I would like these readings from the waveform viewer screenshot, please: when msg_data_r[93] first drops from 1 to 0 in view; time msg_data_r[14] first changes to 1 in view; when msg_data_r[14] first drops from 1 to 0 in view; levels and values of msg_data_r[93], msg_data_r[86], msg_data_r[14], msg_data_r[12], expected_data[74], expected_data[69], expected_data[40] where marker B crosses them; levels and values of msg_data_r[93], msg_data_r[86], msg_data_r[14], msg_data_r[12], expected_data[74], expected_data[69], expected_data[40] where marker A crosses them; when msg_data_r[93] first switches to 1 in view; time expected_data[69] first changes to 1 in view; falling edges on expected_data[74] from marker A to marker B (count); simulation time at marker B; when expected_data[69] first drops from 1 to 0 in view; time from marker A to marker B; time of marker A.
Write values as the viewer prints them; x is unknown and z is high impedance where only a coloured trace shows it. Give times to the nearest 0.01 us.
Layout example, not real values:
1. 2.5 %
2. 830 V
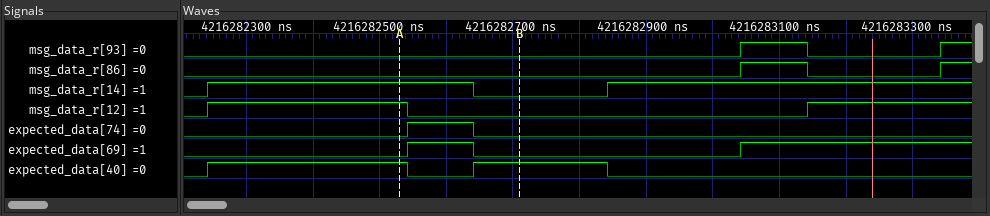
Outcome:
1. 4216283.14 us
2. 4216282.24 us
3. 4216282.64 us
4. msg_data_r[93]=0, msg_data_r[86]=0, msg_data_r[14]=0, msg_data_r[12]=0, expected_data[74]=0, expected_data[69]=0, expected_data[40]=1
5. msg_data_r[93]=0, msg_data_r[86]=0, msg_data_r[14]=1, msg_data_r[12]=1, expected_data[74]=0, expected_data[69]=0, expected_data[40]=1
6. 4216283.04 us
7. 4216282.54 us
8. 1
9. 4216282.71 us
10. 4216282.64 us
11. 0.18 us
12. 4216282.53 us
